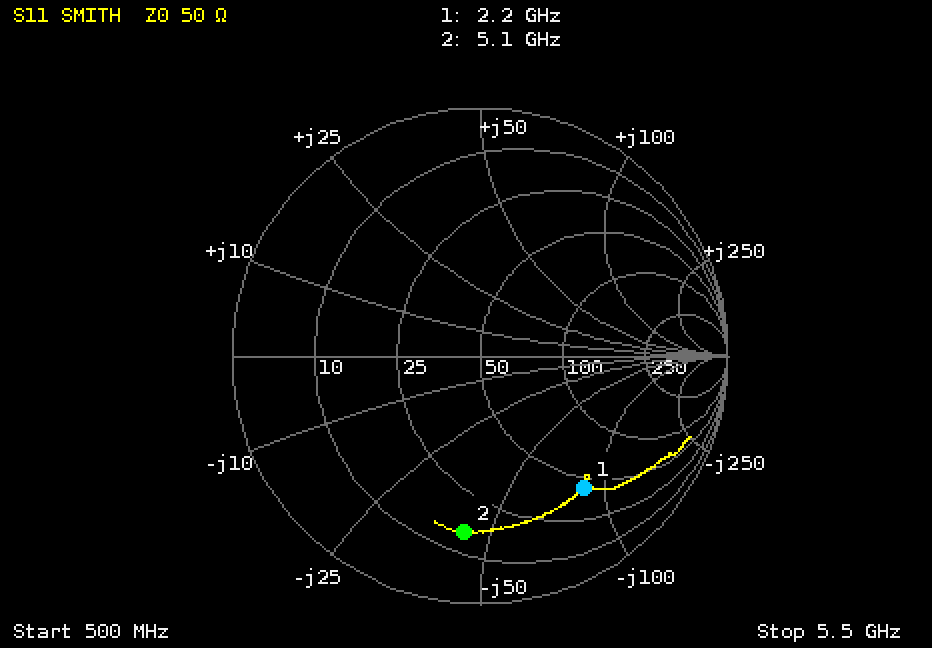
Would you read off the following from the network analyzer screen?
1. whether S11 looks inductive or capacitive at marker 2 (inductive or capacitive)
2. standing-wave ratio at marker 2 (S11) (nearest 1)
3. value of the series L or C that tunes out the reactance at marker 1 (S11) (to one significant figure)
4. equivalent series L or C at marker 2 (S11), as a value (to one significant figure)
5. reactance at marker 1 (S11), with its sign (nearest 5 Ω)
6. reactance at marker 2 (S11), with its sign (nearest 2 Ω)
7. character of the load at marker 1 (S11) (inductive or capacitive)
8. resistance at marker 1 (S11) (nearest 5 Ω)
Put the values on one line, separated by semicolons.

capacitive; 6; 6 nH; 700 fF; -85 Ω; -44 Ω; capacitive; 45 Ω
